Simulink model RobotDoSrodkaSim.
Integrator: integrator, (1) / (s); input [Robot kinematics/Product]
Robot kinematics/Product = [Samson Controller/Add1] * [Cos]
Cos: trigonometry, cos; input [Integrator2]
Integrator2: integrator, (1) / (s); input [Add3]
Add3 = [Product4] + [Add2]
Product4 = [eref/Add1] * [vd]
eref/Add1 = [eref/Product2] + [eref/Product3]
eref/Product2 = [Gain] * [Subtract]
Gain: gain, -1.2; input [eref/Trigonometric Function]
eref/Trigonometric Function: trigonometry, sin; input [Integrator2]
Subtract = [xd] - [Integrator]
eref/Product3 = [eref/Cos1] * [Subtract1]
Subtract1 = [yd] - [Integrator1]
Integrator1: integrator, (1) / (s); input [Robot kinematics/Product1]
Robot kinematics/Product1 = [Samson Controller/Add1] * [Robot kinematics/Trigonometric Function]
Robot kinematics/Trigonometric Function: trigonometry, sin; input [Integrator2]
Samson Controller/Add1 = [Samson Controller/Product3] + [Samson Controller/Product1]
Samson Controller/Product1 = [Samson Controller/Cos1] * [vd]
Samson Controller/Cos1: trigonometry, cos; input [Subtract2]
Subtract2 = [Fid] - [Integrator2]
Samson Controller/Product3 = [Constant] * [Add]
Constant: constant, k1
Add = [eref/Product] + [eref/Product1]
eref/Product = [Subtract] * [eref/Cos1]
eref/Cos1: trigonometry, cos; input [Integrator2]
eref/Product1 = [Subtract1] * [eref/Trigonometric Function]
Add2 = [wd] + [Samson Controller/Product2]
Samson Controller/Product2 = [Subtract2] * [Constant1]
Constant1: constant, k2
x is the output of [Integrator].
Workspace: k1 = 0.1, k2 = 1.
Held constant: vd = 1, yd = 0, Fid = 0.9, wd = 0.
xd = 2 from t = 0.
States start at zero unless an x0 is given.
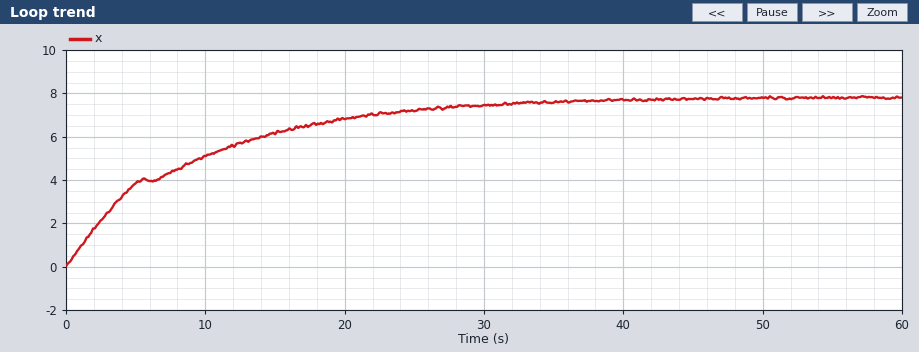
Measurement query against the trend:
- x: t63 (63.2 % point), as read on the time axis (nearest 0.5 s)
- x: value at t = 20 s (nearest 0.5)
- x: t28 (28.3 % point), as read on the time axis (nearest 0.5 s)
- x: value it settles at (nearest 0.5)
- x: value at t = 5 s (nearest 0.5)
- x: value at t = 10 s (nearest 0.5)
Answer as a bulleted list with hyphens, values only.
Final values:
- 9.5 s
- 7.0
- 2.5 s
- 8.0
- 4.0
- 5.0
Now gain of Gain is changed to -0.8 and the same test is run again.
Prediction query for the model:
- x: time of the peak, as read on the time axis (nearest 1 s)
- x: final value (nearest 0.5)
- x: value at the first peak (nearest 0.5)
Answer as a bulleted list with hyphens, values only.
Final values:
- 7 s
- 2.5
- 4.5
